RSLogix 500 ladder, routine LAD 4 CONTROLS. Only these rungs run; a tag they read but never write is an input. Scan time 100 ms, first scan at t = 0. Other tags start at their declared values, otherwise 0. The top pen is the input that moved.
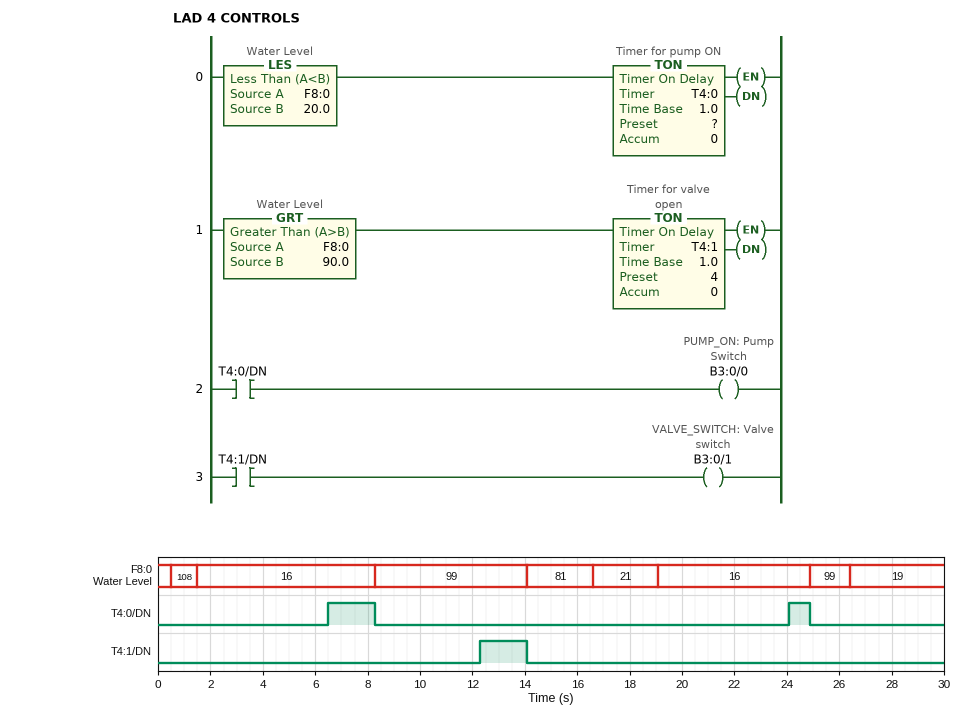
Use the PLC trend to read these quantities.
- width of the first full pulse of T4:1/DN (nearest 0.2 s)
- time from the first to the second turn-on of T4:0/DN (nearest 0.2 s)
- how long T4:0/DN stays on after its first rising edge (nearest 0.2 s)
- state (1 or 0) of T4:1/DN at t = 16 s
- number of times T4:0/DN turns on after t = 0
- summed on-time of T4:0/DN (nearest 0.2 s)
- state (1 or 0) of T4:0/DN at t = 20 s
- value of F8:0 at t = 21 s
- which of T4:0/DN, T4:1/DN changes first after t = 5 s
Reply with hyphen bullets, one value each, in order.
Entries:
- 1.8 s
- 17.6 s
- 1.8 s
- 0
- 2
- 2.6 s
- 0
- 16
- T4:0/DN
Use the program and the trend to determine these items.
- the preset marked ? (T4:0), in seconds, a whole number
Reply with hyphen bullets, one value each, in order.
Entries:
- 5 s
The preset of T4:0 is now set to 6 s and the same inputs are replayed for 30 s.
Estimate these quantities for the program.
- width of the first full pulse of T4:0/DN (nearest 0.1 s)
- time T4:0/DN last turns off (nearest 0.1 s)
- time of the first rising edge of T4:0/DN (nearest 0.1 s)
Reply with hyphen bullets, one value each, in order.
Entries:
- 0.8 s
- 8.3 s
- 7.5 s
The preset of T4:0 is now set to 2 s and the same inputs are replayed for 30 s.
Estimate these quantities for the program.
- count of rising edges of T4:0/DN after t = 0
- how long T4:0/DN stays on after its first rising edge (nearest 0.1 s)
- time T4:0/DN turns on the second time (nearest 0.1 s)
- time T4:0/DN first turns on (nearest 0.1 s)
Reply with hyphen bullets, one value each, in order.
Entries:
- 3
- 4.8 s
- 21.1 s
- 3.5 s
